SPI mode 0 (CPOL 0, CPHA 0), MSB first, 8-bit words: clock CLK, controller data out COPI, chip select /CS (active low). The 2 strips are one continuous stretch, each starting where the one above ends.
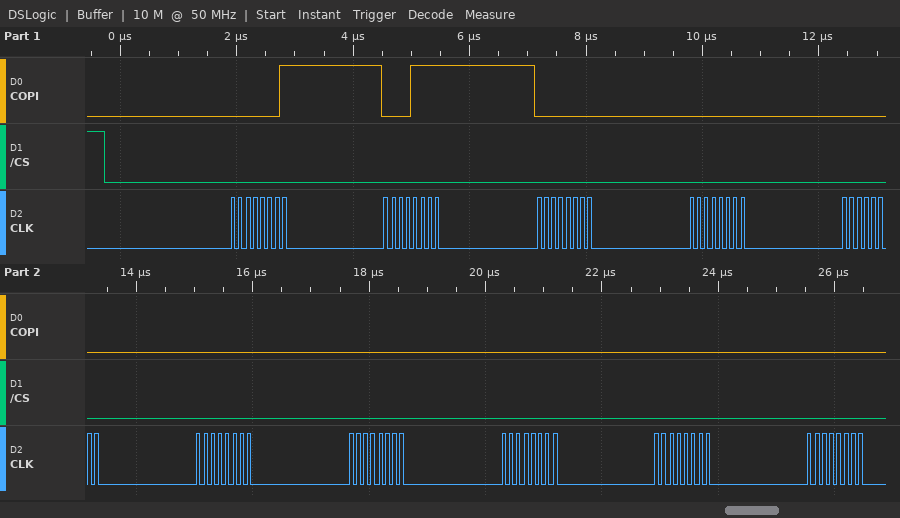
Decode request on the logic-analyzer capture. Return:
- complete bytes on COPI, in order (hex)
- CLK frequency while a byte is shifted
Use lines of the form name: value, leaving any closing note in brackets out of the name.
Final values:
complete bytes on COPI, in order: 01 0F 00 00 00 00 00 00 00 00
CLK frequency while a byte is shifted: 8 MHz
